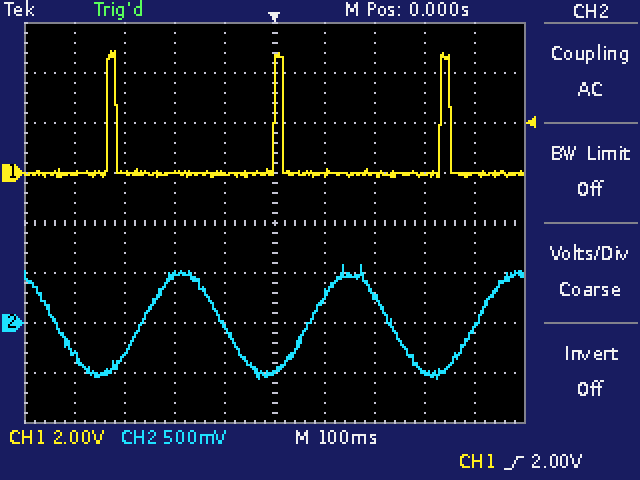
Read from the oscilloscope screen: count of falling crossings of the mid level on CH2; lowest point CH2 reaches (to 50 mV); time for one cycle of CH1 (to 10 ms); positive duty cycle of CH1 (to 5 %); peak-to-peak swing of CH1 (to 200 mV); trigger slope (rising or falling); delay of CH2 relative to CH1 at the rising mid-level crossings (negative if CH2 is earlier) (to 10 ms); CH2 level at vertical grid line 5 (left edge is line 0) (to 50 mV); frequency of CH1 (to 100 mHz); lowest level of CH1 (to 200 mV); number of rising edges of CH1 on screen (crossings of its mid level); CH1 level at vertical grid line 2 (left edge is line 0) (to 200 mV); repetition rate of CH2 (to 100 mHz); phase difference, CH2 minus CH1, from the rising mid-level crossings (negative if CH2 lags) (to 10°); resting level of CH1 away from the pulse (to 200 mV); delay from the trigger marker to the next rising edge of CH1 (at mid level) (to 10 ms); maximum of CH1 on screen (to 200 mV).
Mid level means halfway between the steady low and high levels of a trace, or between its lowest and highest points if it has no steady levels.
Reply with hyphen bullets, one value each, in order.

- 3
- -550 mV
- 330 ms
- 5 %
- 5.0 V
- rising
- +70 ms
- -500 mV
- 3.0 Hz
- -200 mV
- 3
- 0.0 V
- 3.0 Hz
- -80°
- 0.0 V
- 330 ms
- 4.8 V
